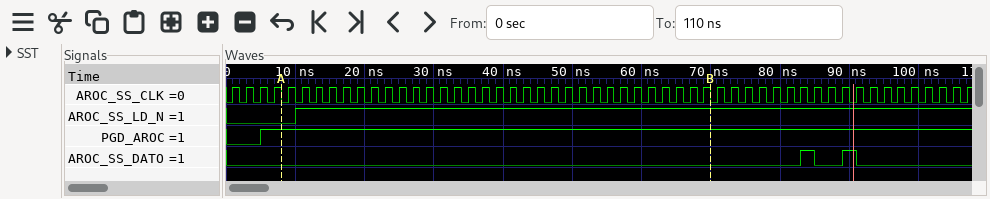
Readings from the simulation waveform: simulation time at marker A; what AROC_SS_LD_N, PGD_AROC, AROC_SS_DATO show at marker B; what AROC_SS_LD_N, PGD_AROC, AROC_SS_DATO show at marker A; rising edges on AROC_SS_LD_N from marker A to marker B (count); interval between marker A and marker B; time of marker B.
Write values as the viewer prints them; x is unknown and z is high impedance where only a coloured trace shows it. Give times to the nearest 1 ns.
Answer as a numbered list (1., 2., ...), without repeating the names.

1. 8 ns
2. AROC_SS_LD_N=1, PGD_AROC=1, AROC_SS_DATO=0
3. AROC_SS_LD_N=0, PGD_AROC=1, AROC_SS_DATO=0
4. 1
5. 62 ns
6. 70 ns
